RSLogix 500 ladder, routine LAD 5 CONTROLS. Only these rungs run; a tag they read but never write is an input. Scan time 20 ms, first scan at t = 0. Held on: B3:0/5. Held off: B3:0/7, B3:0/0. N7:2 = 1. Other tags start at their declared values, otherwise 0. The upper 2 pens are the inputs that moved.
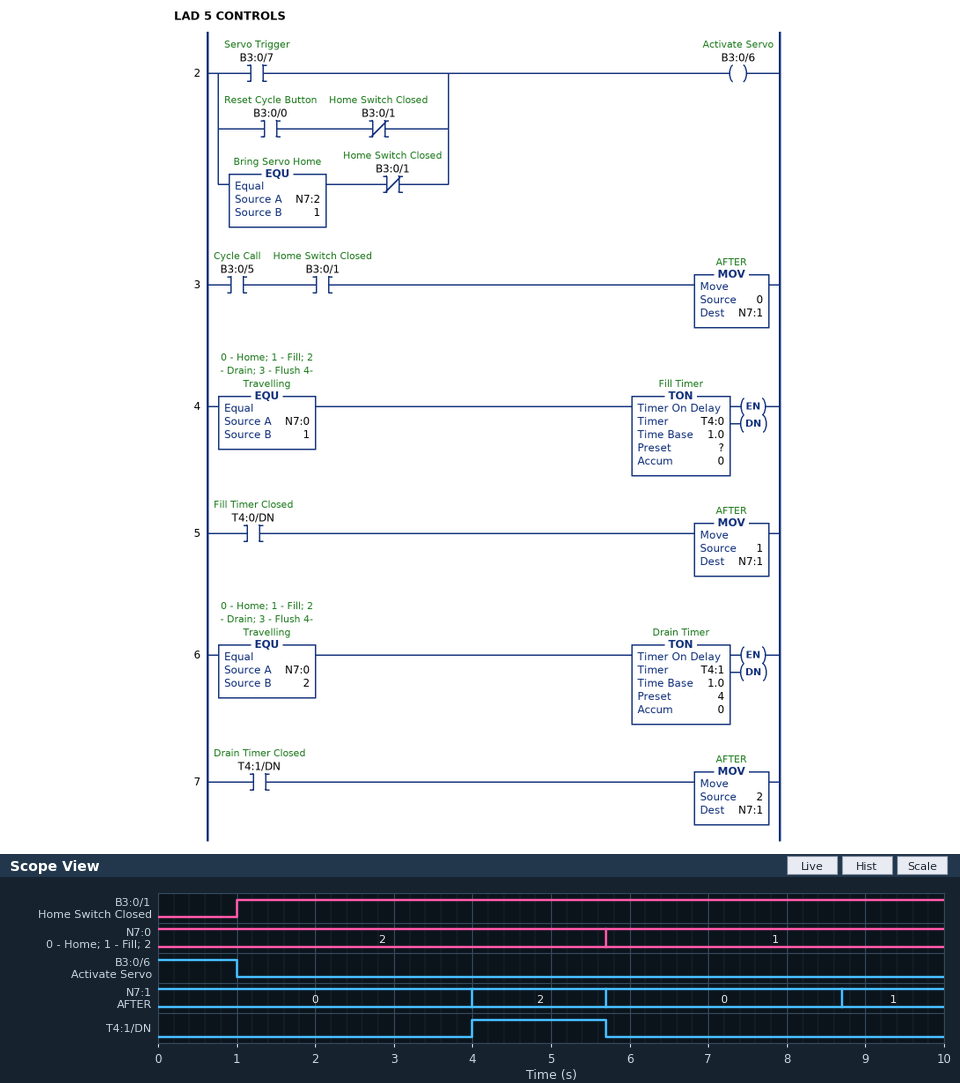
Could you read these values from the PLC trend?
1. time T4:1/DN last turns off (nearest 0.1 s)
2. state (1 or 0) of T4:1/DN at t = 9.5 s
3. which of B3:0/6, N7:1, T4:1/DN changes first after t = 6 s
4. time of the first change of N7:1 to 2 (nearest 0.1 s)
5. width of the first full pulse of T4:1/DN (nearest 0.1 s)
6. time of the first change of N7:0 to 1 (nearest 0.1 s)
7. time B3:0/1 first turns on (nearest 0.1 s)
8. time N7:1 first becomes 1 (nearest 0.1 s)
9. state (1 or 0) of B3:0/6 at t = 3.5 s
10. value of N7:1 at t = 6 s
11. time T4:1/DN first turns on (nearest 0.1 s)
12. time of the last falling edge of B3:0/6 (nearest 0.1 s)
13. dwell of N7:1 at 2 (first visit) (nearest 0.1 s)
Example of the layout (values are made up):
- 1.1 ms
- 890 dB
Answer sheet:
- 5.7 s
- 0
- N7:1
- 4.0 s
- 1.7 s
- 5.7 s
- 1.0 s
- 8.7 s
- 0
- 0
- 4.0 s
- 1.0 s
- 1.7 s
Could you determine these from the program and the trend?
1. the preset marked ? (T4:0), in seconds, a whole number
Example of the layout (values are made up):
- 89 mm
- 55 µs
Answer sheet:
- 3 s
